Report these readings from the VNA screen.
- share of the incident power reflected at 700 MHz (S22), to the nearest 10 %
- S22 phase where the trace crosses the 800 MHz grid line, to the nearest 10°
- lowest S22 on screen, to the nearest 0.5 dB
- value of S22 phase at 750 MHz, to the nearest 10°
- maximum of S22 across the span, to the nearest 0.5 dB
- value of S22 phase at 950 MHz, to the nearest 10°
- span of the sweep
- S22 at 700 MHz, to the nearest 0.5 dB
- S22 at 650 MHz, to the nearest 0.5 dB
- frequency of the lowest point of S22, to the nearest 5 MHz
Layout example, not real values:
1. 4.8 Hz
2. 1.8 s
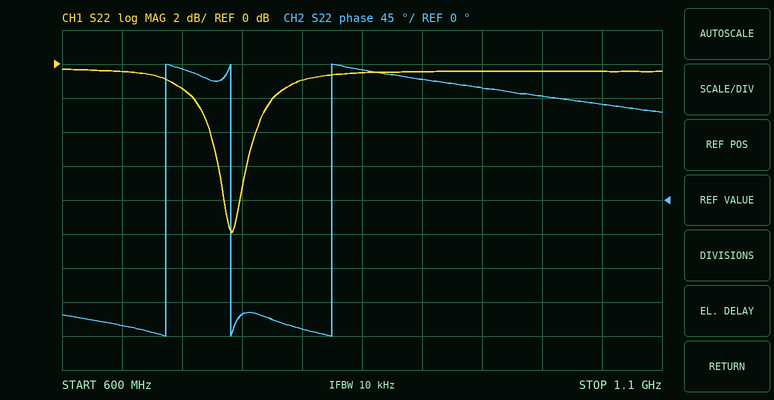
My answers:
1. 70 %
2. -170°
3. -10.0 dB
4. -150°
5. -0.5 dB
6. 150°
7. 500 MHz
8. -1.5 dB
9. -0.5 dB
10. 740 MHz
